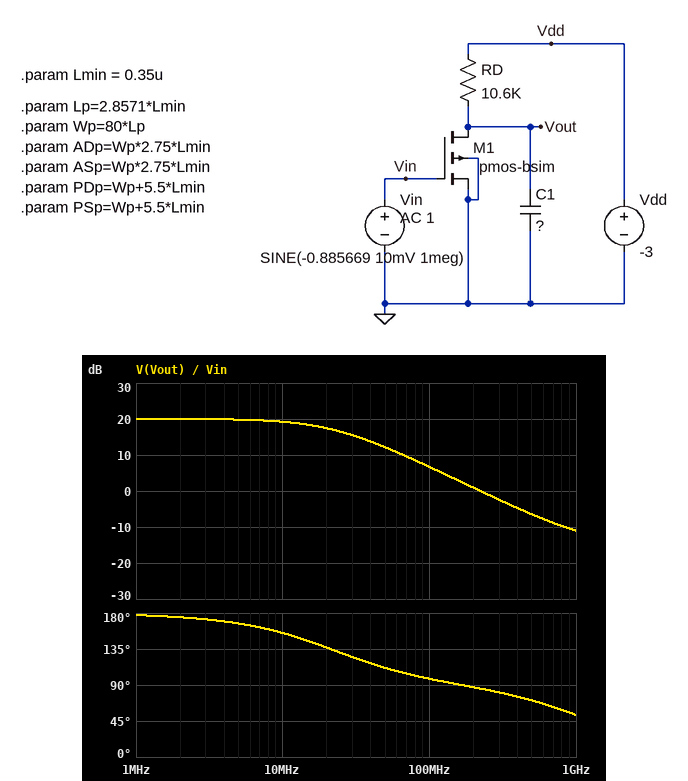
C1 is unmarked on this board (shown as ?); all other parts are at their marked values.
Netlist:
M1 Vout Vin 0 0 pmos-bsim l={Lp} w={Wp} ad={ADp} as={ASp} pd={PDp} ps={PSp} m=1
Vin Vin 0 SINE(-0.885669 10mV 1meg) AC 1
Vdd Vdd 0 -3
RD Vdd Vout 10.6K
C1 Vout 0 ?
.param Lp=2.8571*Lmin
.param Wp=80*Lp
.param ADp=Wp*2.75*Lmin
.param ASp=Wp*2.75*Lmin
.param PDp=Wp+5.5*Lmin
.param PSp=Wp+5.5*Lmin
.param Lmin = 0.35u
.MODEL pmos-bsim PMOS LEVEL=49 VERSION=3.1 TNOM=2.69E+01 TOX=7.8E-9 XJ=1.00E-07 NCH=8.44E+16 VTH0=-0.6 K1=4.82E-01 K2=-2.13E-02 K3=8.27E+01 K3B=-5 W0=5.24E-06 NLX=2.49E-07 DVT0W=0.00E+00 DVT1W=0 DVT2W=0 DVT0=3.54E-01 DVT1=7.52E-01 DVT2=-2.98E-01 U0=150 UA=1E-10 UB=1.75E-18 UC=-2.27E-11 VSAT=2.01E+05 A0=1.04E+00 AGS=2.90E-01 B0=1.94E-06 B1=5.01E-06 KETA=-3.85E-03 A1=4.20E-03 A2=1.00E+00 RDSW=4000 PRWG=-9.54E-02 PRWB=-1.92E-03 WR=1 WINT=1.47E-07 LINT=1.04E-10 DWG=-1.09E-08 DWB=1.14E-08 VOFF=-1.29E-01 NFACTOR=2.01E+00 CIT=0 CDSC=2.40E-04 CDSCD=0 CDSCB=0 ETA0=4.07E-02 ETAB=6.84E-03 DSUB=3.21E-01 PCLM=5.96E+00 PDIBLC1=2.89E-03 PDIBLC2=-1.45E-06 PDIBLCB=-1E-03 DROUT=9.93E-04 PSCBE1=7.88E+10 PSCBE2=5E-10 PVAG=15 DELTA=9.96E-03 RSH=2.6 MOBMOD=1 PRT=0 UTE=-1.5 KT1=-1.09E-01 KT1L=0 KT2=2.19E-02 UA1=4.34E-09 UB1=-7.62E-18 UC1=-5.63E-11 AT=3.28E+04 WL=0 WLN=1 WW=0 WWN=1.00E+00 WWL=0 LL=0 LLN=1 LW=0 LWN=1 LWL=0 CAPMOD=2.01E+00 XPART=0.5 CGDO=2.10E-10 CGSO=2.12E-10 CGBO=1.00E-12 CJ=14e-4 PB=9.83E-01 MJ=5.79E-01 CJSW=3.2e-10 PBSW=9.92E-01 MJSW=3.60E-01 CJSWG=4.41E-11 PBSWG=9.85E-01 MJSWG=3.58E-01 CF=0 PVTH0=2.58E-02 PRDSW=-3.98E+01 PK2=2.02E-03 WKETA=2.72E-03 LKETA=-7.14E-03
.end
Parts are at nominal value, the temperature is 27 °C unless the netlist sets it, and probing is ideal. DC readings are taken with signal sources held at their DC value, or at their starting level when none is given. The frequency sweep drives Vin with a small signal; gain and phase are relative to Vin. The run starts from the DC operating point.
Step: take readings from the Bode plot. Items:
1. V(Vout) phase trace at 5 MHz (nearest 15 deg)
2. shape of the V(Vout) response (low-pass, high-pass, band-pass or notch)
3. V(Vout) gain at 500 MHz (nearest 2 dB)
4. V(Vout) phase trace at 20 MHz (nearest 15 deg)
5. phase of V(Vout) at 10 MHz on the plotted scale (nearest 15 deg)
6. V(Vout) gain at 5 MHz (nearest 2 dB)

165 deg
low-pass
-6 dB
135 deg
150 deg
20 dB
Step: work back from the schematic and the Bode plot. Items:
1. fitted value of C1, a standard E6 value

680 fF
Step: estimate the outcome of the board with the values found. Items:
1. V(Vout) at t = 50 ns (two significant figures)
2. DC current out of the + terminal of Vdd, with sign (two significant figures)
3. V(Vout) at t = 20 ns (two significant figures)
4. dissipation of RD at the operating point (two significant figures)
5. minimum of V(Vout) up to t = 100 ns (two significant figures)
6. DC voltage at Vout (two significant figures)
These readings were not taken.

-1.5 V
-140 µA
-1.5 V
210 µW
-1.6 V
-1.5 V
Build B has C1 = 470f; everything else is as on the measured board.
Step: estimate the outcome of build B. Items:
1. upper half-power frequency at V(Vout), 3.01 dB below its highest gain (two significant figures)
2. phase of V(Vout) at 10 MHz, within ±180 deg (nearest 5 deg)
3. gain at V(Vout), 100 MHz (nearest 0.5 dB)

30 MHz
160 deg
9.5 dB
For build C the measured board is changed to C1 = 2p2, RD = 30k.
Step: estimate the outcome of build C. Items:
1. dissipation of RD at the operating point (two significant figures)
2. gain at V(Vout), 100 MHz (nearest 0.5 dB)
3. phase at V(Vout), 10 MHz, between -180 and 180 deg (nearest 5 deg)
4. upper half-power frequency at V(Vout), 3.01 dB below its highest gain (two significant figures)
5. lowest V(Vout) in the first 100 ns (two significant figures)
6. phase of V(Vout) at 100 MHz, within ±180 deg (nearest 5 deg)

270 µW
-9.0 dB
160 deg
30 MHz
-140 mV
95 deg
